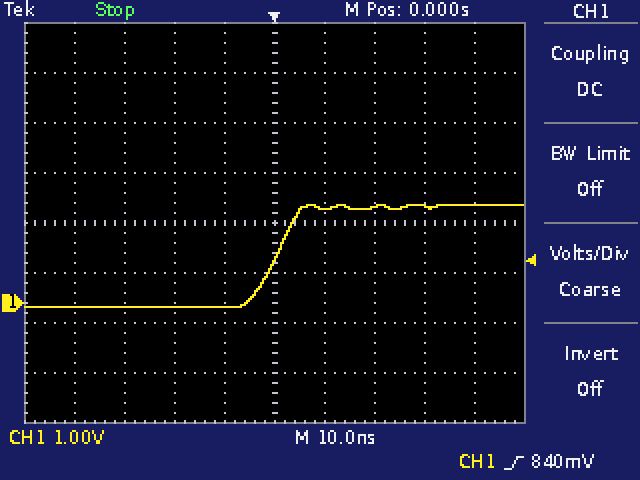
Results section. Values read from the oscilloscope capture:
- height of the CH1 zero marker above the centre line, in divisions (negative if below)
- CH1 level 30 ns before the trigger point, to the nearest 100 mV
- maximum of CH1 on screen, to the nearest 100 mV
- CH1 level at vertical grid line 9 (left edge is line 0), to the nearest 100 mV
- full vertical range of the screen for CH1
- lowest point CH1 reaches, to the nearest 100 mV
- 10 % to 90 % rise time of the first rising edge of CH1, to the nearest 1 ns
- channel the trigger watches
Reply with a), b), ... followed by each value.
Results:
a) -1.6 div
b) -100 mV
c) 2.0 V
d) 2.0 V
e) 8 V
f) -100 mV
g) 9 ns
h) CH1
